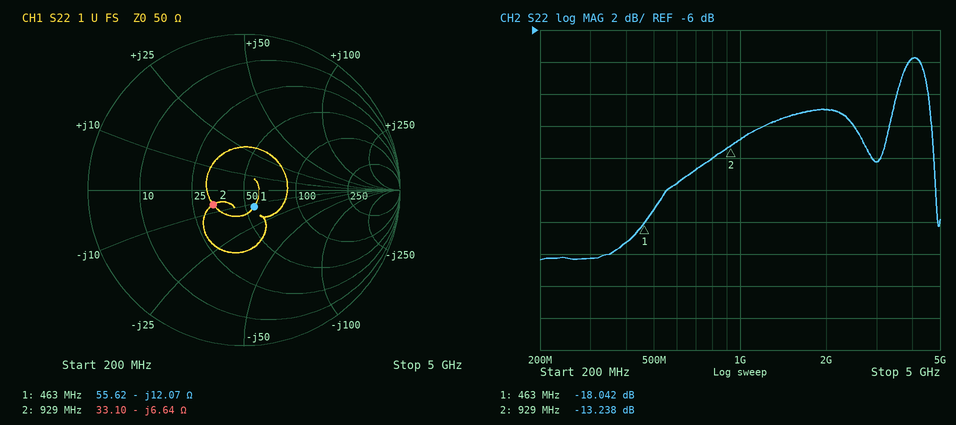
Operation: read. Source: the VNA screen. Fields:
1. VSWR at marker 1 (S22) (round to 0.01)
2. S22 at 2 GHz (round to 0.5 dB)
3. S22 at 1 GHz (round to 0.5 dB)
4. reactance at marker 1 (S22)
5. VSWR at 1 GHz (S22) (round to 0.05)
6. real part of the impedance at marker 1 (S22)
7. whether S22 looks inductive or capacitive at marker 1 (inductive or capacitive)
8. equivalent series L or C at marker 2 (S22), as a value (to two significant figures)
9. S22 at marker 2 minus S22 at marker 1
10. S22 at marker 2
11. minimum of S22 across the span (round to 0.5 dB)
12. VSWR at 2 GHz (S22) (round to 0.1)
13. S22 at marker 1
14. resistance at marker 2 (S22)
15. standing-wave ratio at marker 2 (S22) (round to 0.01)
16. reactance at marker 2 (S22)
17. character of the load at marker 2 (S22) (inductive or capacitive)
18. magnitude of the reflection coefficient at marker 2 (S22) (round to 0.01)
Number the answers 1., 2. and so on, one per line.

1. 1.29
2. -11.0 dB
3. -13.0 dB
4. -12.07 Ω
5. 1.60
6. 55.62 Ω
7. capacitive
8. 26 pF
9. 4.804 dB
10. -13.238 dB
11. -20.5 dB
12. 1.8
13. -18.042 dB
14. 33.10 Ω
15. 1.56
16. -6.64 Ω
17. capacitive
18. 0.22
